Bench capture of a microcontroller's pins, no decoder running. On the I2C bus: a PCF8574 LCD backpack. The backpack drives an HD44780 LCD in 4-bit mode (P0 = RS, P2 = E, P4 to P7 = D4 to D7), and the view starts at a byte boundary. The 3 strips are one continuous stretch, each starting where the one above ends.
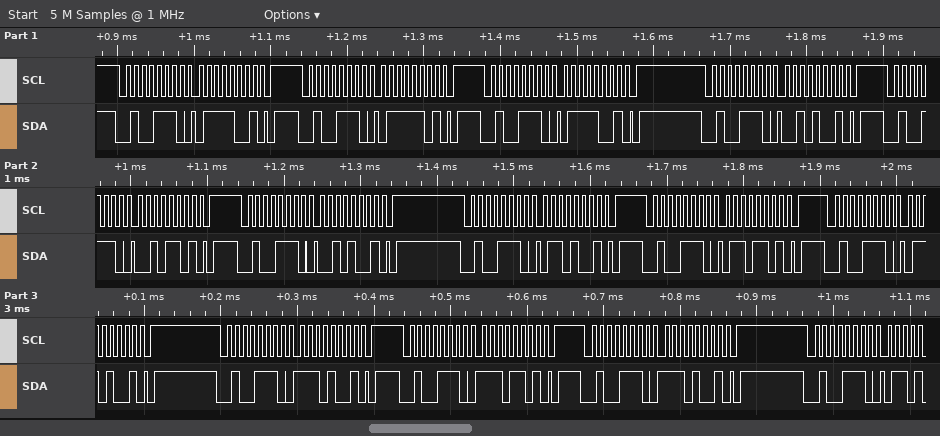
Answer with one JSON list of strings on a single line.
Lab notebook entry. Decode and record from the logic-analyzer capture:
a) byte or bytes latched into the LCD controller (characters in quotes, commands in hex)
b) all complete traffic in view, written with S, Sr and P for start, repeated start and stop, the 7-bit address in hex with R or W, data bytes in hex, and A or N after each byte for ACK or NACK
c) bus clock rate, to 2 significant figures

["'r' 'n'", "S 27W A 79 A P S 27W A 7D A P S 27W A 79 A P S 27W A 29 A P S 27W A 2D A P S 27W A 29 A P S 27W A 69 A P S 27W A 6D A P S 27W A 69 A P S 27W A E9 A P S 27W A ED A P S 27W A E9 A P S 27W A", "100 kHz"]
